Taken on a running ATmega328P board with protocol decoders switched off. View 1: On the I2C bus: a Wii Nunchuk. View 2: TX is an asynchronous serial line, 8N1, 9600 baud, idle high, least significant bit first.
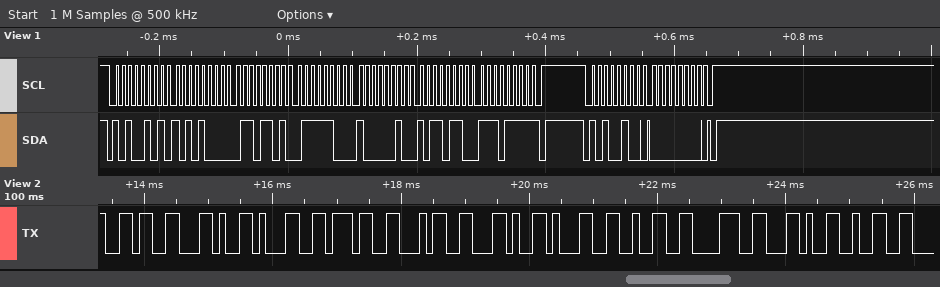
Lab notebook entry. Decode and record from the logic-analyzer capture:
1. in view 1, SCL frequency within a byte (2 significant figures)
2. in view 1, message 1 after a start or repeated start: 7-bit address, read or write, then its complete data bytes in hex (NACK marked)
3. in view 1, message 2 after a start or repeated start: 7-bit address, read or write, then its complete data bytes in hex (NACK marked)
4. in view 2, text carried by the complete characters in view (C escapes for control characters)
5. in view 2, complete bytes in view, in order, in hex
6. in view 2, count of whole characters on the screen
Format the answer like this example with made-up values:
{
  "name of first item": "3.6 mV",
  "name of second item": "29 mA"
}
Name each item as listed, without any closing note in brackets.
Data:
{
  "in view 1, SCL frequency within a byte": "100 kHz",
  "in view 1, message 1 after a start or repeated start: 7-bit address, read or write, then its complete data bytes in hex": "0x52 read: A8 6D 7C 82 B6 EF NACK",
  "in view 1, message 2 after a start or repeated start: 7-bit address, read or write, then its complete data bytes in hex": "0x52 write: 00",
  "in view 2, text carried by the complete characters in view": "\"6,174,128,2\"",
  "in view 2, complete bytes in view, in order, in hex": "36 2C 31 37 34 2C 31 32 38 2C 32",
  "in view 2, count of whole characters on the screen": "11"
}
